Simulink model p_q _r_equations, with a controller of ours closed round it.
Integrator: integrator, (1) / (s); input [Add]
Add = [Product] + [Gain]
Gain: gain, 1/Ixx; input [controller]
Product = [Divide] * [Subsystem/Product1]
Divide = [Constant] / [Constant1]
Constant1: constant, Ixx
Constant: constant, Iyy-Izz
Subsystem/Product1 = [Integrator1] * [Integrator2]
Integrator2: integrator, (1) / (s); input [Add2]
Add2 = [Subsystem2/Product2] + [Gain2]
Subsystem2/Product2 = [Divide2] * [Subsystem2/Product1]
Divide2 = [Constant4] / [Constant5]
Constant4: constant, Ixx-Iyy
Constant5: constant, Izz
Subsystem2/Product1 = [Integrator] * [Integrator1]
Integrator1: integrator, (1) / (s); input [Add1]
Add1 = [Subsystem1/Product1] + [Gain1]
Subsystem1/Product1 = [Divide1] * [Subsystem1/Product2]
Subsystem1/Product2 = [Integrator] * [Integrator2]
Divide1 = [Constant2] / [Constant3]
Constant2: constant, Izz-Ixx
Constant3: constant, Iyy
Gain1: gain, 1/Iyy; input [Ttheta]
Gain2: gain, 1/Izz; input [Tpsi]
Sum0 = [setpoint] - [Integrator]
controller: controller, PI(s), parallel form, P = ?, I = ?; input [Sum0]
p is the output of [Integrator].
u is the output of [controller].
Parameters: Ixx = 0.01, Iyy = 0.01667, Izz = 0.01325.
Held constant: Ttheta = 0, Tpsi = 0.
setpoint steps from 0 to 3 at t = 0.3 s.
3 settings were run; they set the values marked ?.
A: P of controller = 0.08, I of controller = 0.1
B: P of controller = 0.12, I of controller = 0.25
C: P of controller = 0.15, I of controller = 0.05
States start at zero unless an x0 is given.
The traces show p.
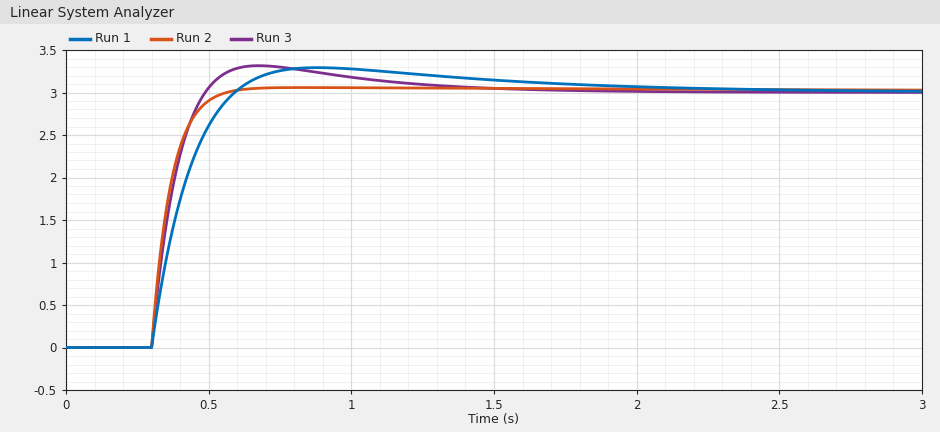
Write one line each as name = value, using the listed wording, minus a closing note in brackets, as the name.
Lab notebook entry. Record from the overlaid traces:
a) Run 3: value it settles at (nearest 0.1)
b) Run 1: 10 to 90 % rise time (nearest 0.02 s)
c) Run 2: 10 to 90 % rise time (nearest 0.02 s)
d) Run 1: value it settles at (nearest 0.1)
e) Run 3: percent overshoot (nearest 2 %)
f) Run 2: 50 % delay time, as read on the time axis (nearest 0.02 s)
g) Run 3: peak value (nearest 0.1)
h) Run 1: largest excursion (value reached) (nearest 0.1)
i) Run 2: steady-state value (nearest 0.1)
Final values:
Run 3: value it settles at = 3.0
Run 1: 10 to 90 % rise time = 0.20 s
Run 2: 10 to 90 % rise time = 0.14 s
Run 1: value it settles at = 3.0
Run 3: percent overshoot = 10 %
Run 2: 50 % delay time, as read on the time axis = 0.34 s
Run 3: peak value = 3.3
Run 1: largest excursion (value reached) = 3.3
Run 2: steady-state value = 3.0
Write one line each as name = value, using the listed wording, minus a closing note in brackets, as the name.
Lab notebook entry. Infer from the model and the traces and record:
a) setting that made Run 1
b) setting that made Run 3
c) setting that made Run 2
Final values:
setting that made Run 1 = A
setting that made Run 3 = B
setting that made Run 2 = C
